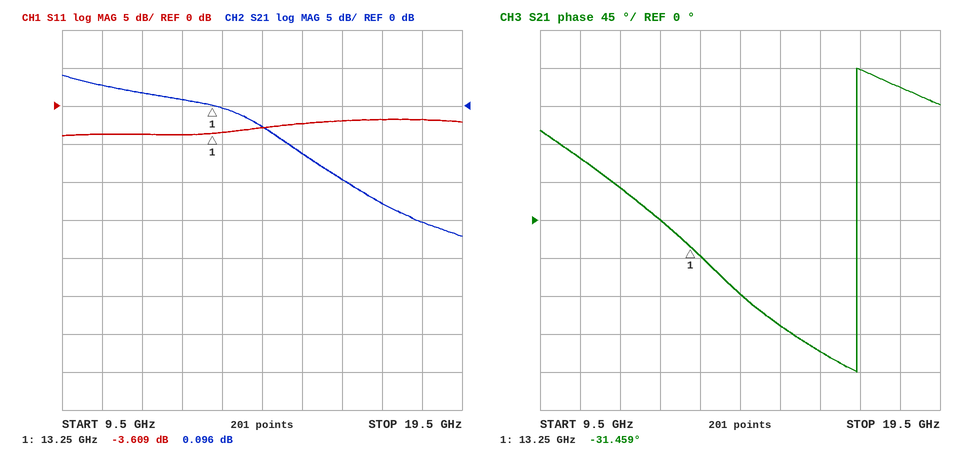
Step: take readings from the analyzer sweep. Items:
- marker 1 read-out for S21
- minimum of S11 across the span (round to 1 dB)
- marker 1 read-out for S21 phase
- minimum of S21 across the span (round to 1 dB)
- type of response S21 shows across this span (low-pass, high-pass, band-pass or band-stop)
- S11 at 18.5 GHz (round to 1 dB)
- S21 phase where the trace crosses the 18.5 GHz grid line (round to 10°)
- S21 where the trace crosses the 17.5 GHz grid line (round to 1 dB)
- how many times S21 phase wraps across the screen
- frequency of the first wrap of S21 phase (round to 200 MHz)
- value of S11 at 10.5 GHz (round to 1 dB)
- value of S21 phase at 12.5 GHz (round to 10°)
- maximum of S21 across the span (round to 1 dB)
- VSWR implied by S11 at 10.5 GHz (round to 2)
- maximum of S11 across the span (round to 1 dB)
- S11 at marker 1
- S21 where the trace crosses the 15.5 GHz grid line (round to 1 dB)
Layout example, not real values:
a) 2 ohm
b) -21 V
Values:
a) 0.096 dB
b) -4 dB
c) -31.459°
d) -17 dB
e) low-pass
f) -2 dB
g) 160°
h) -13 dB
i) 1
j) 17.4 GHz
k) -4 dB
l) 0°
m) 4 dB
n) 4
o) -2 dB
p) -3.609 dB
q) -6 dB
